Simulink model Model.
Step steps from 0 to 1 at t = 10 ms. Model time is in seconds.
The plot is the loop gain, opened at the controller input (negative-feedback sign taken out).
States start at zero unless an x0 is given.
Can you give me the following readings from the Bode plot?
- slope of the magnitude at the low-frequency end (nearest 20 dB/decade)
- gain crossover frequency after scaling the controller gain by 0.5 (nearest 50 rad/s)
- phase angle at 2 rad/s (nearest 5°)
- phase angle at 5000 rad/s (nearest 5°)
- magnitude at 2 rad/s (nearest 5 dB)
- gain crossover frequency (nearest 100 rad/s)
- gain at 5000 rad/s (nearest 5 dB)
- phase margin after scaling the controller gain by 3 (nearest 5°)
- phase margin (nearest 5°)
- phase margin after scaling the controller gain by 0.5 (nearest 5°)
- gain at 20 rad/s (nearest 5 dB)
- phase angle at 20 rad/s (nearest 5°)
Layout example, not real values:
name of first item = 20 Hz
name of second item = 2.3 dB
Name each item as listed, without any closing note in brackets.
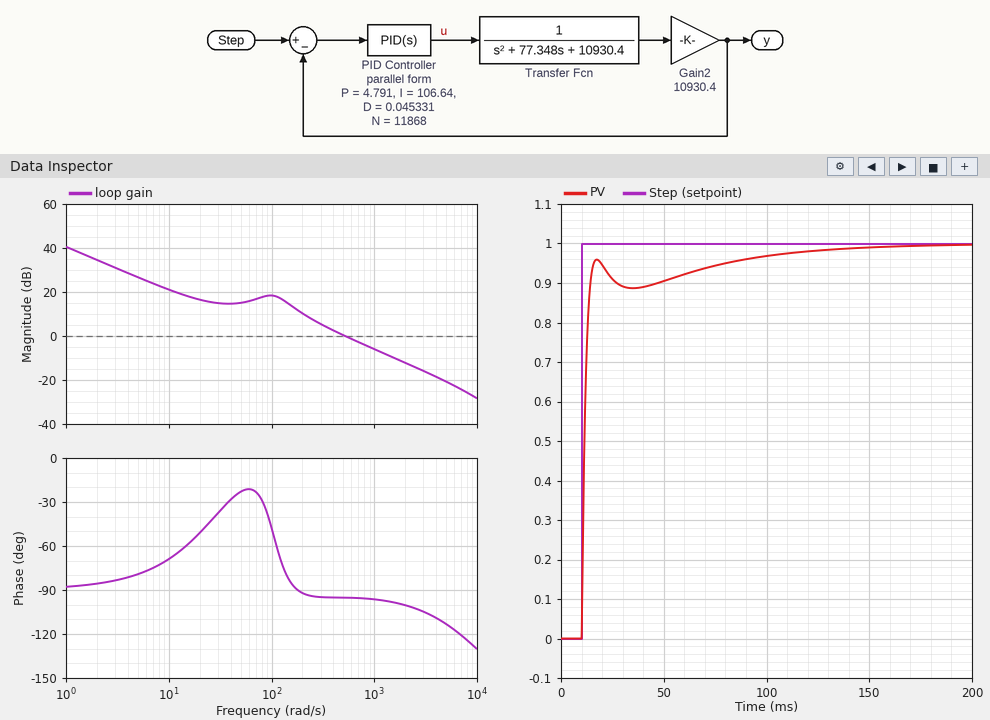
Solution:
slope of the magnitude at the low-frequency end = -20 dB/decade
gain crossover frequency after scaling the controller gain by 0.5 = 300 rad/s
phase angle at 2 rad/s = -85°
phase angle at 5000 rad/s = -115°
magnitude at 2 rad/s = 35 dB
gain crossover frequency = 500 rad/s
gain at 5000 rad/s = -20 dB
phase margin after scaling the controller gain by 3 = 80°
phase margin = 85°
phase margin after scaling the controller gain by 0.5 = 85°
gain at 20 rad/s = 15 dB
phase angle at 20 rad/s = -50°
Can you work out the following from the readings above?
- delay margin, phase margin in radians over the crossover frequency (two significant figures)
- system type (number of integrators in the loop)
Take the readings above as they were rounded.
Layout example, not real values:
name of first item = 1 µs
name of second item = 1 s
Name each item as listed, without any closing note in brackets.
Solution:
delay margin, phase margin in radians over the crossover frequency = 0.0030 s
system type = 1
